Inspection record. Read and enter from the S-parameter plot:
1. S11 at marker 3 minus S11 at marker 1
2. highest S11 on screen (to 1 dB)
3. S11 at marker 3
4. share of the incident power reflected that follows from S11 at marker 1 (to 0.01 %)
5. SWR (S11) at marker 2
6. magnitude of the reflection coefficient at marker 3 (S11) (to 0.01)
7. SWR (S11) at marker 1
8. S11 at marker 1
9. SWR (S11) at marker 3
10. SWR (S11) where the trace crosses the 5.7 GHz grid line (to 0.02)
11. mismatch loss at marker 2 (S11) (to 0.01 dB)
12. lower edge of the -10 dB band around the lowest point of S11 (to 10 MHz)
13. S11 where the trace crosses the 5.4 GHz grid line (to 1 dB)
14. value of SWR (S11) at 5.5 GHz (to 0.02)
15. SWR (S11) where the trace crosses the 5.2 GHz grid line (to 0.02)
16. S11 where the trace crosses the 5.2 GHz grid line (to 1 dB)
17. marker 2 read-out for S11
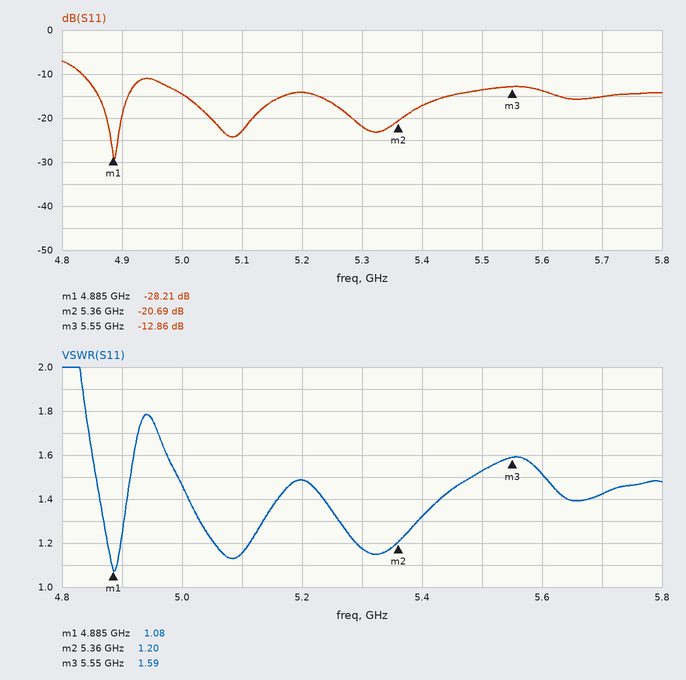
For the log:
15.35 dB
-7 dB
-12.86 dB
0.15 %
1.20
0.23
1.08
-28.21 dB
1.59
1.42
0.04 dB
4.83 GHz
-17 dB
1.52
1.48
-14 dB
-20.69 dB
